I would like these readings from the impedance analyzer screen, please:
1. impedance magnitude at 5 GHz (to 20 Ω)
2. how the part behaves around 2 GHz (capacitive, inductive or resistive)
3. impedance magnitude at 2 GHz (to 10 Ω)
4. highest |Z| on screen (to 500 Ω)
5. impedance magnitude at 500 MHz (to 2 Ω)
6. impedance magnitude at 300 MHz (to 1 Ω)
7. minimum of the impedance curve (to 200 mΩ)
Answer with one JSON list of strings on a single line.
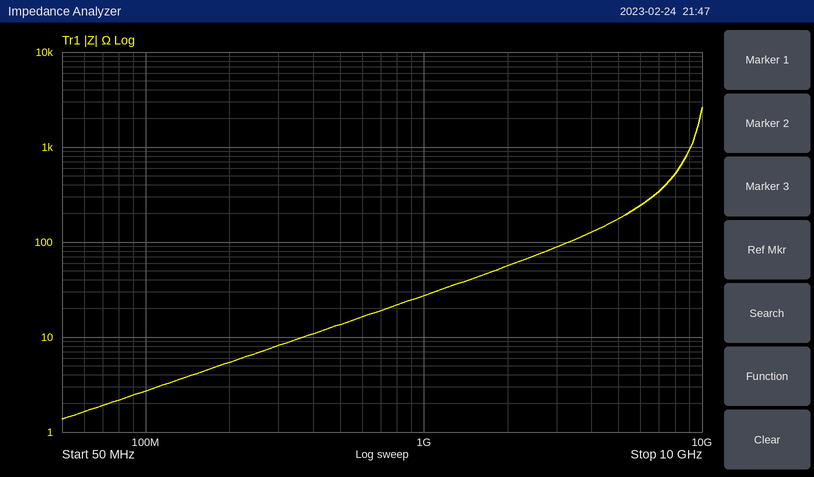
["180 Ω", "inductive", "60 Ω", "2.5 kΩ", "14 Ω", "8 Ω", "1.4 Ω"]
